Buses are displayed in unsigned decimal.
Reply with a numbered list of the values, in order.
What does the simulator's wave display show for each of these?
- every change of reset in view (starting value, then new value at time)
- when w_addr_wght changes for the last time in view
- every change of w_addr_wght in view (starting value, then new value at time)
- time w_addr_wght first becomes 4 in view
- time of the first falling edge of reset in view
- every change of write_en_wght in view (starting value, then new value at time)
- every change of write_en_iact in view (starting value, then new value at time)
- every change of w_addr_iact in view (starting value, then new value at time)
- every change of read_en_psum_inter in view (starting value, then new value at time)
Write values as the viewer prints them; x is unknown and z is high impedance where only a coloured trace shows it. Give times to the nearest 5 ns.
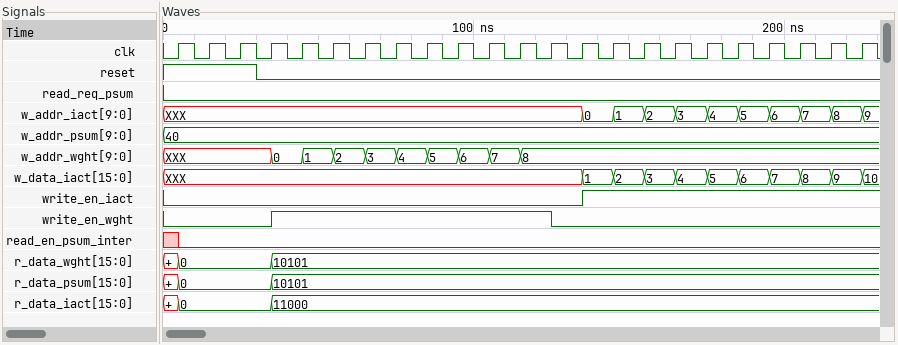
1. 1, 0 at 30 ns
2. 115 ns
3. XXX, 0 at 35 ns, 1 at 45 ns, 2 at 55 ns, 3 at 65 ns, 4 at 75 ns, 5 at 85 ns, 6 at 95 ns, 7 at 105 ns, 8 at 115 ns
4. 75 ns
5. 30 ns
6. 0, 1 at 35 ns, 0 at 125 ns
7. 0, 1 at 135 ns
8. XXX, 0 at 135 ns, 1 at 145 ns, 2 at 155 ns, 3 at 165 ns, 4 at 175 ns, 5 at 185 ns, 6 at 195 ns, 7 at 205 ns, 8 at 215 ns, 9 at 225 ns
9. x, 0 at 5 ns
